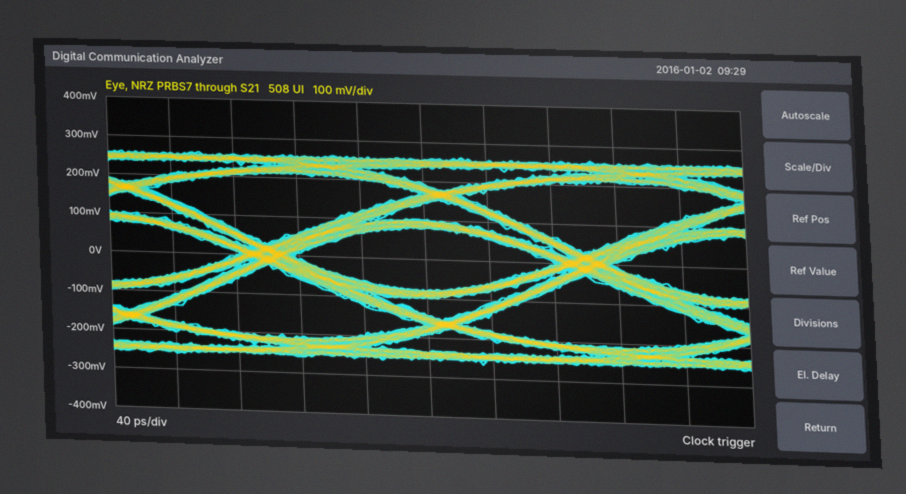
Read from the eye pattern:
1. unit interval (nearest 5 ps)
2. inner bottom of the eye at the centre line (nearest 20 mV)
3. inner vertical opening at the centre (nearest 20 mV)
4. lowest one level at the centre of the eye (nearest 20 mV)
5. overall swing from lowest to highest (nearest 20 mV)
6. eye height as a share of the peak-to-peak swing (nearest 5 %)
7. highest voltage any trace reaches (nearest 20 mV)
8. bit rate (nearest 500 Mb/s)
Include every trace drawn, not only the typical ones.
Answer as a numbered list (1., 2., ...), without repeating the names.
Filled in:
1. 200 ps
2. -80 mV
3. 160 mV
4. 80 mV
5. 520 mV
6. 30 %
7. 260 mV
8. 5.0 Gb/s
